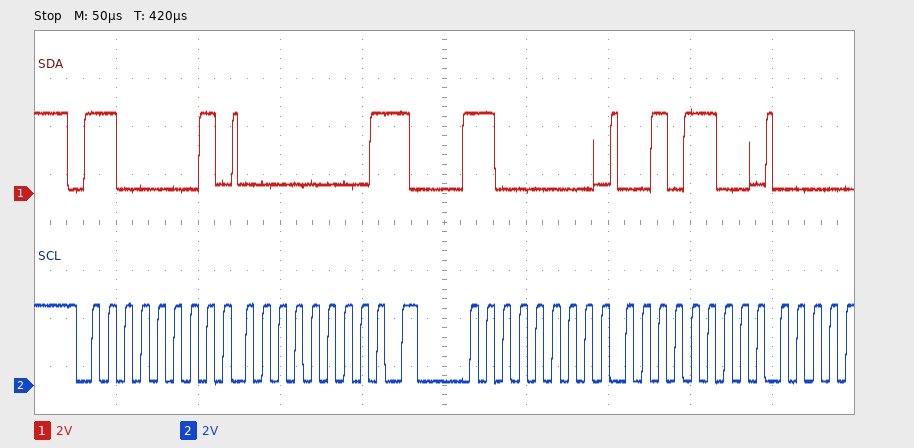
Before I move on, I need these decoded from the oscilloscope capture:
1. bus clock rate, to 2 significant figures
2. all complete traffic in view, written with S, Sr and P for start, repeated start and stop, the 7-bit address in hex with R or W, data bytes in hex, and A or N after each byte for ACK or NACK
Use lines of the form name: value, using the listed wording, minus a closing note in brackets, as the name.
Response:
bus clock rate, to 2 significant figures: 100 kHz
all complete traffic in view, written with S, Sr and P for start, repeated start and stop, the 7-bit address in hex with R or W, data bytes in hex, and A or N after each byte for ACK or NACK: S 60R A 00 N Sr 60W A 2C A
